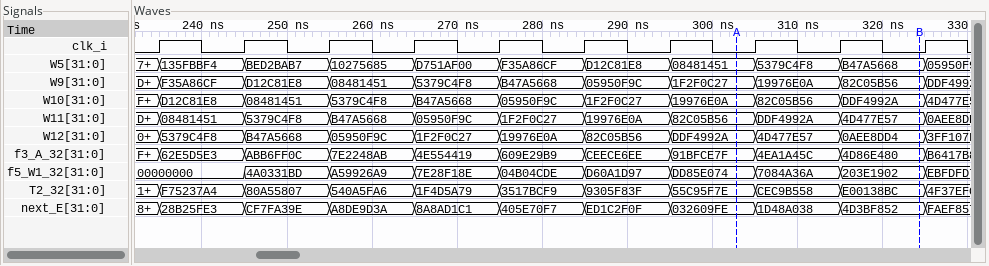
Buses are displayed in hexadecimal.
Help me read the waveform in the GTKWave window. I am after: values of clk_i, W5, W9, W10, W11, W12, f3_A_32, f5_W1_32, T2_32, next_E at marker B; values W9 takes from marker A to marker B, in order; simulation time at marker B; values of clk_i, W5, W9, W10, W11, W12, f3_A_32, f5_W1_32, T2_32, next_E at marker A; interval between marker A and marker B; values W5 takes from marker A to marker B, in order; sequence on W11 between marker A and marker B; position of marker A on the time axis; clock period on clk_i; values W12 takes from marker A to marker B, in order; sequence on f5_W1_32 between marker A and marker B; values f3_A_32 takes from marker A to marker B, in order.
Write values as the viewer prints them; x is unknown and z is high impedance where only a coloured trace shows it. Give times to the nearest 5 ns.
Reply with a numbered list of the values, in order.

1. clk_i=0, W5=B47A5668, W9=82C05B56, W10=DDF4992A, W11=4D477E57, W12=0AEE8DD4, f3_A_32=4D86E480, f5_W1_32=203E1902, T2_32=E00138BC, next_E=4D3BF852
2. 1F2F0C27, 19976E0A, 82C05B56
3. 325 ns
4. clk_i=0, W5=08481451, W9=1F2F0C27, W10=19976E0A, W11=82C05B56, W12=DDF4992A, f3_A_32=91BFCE7F, f5_W1_32=DD85E074, T2_32=55C95F7E, next_E=032609FE
5. 20 ns
6. 08481451, 5379C4F8, B47A5668
7. 82C05B56, DDF4992A, 4D477E57
8. 305 ns
9. 10 ns
10. DDF4992A, 4D477E57, 0AEE8DD4
11. DD85E074, 7084A36A, 203E1902
12. 91BFCE7F, 4EA1A45C, 4D86E480
